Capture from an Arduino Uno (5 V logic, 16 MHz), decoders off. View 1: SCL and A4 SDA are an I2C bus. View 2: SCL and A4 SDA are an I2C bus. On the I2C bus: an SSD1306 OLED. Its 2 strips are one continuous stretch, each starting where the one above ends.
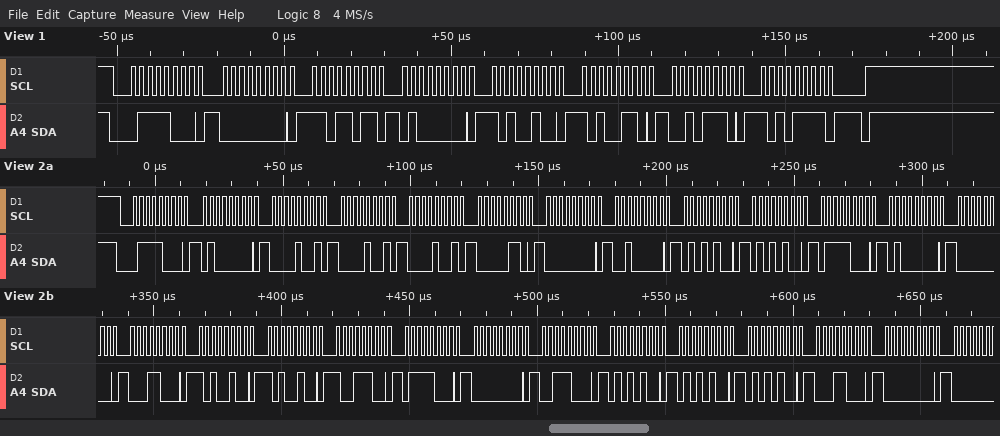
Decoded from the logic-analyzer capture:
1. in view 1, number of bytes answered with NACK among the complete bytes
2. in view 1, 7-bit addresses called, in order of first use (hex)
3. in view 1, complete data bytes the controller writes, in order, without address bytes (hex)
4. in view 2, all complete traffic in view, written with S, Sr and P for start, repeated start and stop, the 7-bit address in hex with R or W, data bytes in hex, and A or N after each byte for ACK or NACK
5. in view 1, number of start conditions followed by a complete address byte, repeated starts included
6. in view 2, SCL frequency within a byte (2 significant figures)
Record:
0
0x3C
00 DB 40 A4 A6 2E AF
S 3CW A 40 A 09 A 09 A 09 A 06 A 00 A 20 A 54 A 54 A 78 A 40 A 00 A 18 A A4 A A4 A 9C A 78 A 00 A 38 A 54 A 54 A 54 A 18 A 00 A
1
400 kHz
